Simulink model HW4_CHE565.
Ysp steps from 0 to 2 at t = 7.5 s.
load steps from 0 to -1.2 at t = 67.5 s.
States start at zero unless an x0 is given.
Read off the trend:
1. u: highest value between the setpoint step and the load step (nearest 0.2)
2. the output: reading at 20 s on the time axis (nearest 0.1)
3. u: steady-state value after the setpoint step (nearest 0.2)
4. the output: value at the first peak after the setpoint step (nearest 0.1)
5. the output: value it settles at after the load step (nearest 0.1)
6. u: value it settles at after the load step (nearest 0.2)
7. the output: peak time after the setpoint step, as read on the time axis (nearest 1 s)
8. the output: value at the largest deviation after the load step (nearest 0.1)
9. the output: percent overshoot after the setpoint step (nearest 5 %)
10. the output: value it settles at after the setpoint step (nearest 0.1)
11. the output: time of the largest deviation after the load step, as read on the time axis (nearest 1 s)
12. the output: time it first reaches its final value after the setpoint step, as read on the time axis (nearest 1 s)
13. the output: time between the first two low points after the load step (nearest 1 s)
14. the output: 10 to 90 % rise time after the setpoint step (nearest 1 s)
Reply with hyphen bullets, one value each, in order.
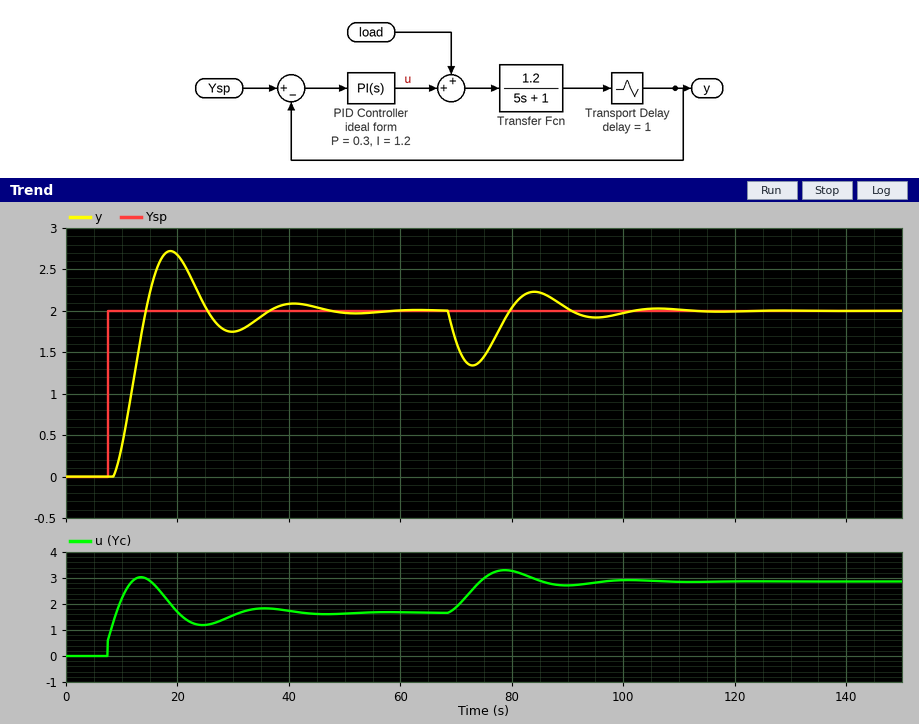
- 3.0
- 2.7
- 1.6
- 2.7
- 2.0
- 2.8
- 19 s
- 1.3
- 35 %
- 2.0
- 73 s
- 14 s
- 22 s
- 4 s
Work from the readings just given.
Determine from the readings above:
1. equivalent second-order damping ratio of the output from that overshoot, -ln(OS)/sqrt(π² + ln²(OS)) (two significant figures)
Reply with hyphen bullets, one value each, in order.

- 0.32
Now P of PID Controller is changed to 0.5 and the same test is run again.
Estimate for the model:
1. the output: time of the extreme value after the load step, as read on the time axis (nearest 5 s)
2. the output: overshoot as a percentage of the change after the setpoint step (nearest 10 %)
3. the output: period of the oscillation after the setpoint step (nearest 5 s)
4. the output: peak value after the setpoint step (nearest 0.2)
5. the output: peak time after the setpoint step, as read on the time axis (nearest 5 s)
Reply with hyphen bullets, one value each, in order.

- 70 s
- 50 %
- 15 s
- 3.0
- 15 s
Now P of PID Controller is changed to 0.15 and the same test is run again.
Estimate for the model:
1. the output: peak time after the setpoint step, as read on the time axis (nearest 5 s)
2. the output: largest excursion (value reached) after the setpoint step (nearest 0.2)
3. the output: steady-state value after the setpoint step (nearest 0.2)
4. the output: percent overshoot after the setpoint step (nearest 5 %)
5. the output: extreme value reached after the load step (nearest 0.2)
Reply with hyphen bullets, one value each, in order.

- 25 s
- 2.4
- 2.0
- 20 %
- 1.2
